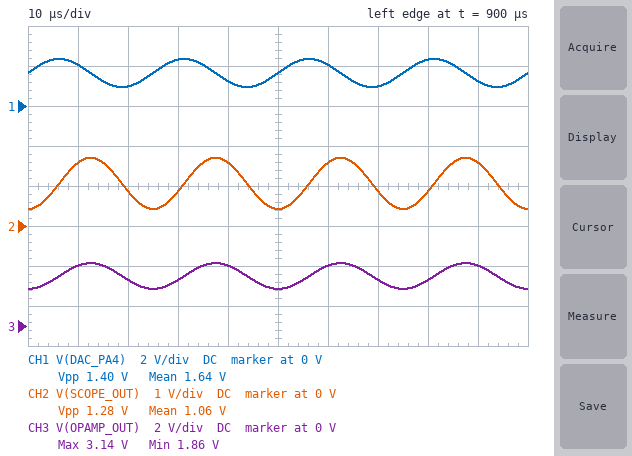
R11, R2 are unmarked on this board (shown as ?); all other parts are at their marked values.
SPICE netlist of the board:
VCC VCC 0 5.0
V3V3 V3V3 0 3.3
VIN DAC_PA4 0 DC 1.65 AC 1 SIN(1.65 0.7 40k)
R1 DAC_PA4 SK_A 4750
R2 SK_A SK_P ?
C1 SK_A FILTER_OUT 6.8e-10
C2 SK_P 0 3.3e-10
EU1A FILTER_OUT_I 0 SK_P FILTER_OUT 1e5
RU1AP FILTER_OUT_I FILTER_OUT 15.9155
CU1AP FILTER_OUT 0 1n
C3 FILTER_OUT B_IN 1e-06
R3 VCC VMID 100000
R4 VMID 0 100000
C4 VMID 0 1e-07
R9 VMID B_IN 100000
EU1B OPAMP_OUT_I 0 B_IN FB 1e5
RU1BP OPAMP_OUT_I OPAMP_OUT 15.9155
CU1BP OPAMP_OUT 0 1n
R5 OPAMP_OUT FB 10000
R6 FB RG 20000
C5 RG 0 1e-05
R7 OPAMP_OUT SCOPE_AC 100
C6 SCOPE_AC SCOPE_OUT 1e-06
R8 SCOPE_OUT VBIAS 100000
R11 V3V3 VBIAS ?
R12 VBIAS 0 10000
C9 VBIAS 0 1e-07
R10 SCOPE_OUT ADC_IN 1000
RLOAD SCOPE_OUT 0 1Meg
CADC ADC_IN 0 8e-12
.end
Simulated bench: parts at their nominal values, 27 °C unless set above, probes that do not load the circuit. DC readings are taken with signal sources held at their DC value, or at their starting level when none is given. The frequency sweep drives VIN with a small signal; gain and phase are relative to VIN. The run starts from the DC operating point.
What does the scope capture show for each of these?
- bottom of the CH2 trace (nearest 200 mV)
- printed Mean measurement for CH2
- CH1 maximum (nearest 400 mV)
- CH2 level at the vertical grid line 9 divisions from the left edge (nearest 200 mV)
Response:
400 mV
1.06 V
2.4 V
1.6 V
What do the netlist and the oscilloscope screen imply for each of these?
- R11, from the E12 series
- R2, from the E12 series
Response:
18 kΩ
15 kΩ
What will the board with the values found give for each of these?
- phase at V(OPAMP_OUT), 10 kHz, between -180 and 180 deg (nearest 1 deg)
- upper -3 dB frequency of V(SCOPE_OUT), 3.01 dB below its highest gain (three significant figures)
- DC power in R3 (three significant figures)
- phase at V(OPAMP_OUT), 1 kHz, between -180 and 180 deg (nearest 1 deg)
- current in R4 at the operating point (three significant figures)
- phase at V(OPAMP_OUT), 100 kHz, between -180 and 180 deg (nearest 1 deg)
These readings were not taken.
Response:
-24 deg
33.9 kHz
62.5 µW
-2 deg
25.0 µA
-142 deg
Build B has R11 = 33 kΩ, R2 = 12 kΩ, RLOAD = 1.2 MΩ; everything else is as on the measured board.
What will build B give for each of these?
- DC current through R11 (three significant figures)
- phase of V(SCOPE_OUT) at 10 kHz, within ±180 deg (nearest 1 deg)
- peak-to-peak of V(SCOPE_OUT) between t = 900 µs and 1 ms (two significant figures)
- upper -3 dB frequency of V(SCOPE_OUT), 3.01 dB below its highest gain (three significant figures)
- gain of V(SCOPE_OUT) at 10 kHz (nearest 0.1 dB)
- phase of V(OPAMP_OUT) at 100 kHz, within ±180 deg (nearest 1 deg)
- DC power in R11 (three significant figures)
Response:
76.9 µA
-20 deg
1.5 V
40.4 kHz
3.4 dB
-139 deg
195 µW
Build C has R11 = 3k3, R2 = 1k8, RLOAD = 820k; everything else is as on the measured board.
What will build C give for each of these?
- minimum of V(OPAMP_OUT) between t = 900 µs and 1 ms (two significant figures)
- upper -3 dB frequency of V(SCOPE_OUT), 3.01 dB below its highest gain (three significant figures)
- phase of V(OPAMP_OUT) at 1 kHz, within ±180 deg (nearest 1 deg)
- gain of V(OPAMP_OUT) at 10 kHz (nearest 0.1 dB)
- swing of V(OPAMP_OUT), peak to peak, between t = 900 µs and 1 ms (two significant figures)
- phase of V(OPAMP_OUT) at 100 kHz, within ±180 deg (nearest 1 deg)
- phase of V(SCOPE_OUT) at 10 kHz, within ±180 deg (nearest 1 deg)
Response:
1.5 V
103 kHz
-1 deg
3.5 dB
2.0 V
-80 deg
-8 deg
